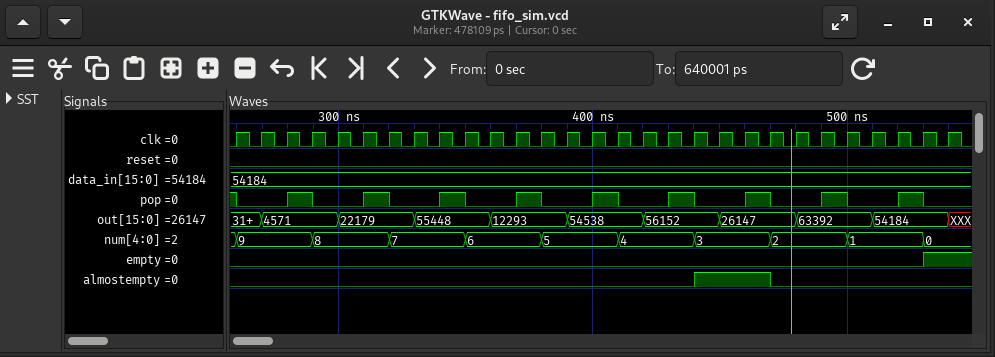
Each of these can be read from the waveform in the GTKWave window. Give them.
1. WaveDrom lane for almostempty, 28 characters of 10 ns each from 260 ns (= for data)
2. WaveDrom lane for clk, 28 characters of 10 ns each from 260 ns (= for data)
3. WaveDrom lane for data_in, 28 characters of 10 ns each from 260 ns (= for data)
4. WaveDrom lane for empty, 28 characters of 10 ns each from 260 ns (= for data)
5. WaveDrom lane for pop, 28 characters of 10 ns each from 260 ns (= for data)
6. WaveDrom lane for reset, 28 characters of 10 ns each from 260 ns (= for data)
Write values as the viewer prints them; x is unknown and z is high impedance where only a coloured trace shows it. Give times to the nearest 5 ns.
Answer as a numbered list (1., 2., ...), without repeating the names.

1. {name: 'almostempty', wave: '0.................1..0......'}
2. {name: 'clk', wave: 'p...........................'}
3. {name: 'data_in', wave: '=...........................', data: '54184'}
4. {name: 'empty', wave: '0..........................1'}
5. {name: 'pop', wave: '0.10.10.10.10.10.10.10.10.10'}
6. {name: 'reset', wave: '0...........................'}
